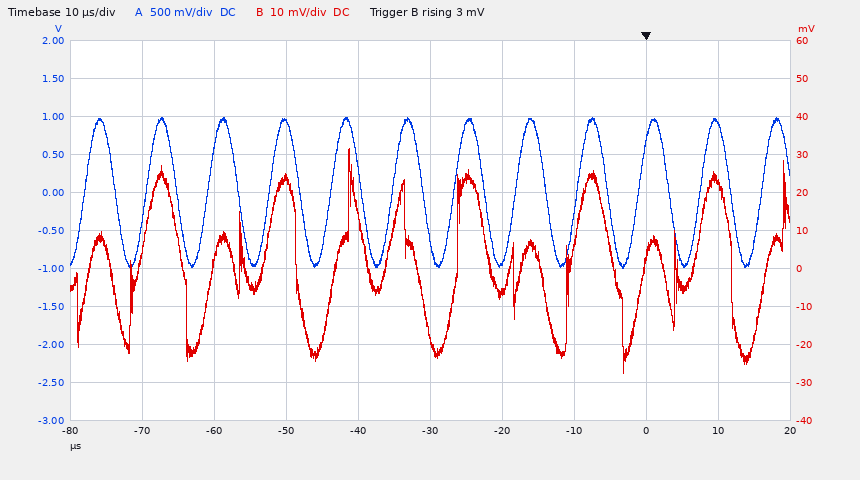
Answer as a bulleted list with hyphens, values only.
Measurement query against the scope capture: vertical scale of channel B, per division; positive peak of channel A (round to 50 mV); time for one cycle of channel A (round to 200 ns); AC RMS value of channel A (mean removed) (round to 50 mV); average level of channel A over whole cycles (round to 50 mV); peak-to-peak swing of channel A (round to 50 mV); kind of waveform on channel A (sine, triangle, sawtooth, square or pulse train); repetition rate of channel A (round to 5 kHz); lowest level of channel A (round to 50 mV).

- 10 mV
- 1.00 V
- 8.6 µs
- 700 mV
- 0 mV
- 2.00 V
- sine
- 115 kHz
- -1.00 V
